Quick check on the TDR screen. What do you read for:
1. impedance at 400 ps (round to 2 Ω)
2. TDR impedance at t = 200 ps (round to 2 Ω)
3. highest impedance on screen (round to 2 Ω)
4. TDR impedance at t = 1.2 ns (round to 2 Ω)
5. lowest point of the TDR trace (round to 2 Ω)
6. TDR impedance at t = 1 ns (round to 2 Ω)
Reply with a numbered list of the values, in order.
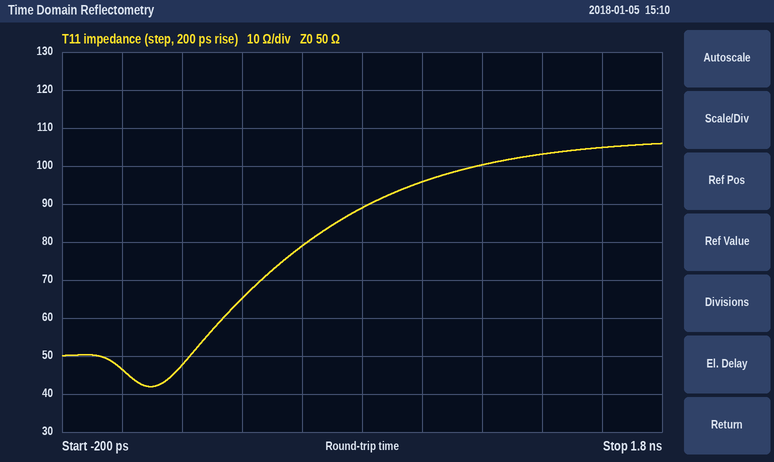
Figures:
1. 66 Ω
2. 48 Ω
3. 106 Ω
4. 100 Ω
5. 42 Ω
6. 96 Ω
